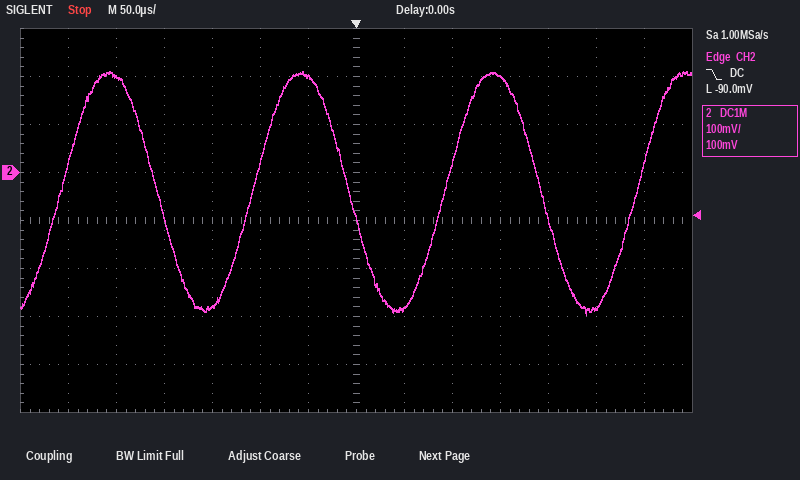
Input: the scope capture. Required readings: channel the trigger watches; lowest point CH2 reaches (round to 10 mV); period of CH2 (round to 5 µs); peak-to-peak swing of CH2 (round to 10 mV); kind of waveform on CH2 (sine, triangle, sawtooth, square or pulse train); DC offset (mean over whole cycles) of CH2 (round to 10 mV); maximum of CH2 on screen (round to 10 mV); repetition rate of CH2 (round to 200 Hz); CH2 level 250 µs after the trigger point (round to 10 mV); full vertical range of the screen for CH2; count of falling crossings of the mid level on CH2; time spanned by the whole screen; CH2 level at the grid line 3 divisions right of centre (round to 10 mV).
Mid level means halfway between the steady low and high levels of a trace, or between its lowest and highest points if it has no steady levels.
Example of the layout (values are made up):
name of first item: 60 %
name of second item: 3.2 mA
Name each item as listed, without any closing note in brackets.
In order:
channel the trigger watches: CH2
lowest point CH2 reaches: -300 mV
period of CH2: 200 µs
peak-to-peak swing of CH2: 510 mV
kind of waveform on CH2: sine
DC offset (mean over whole cycles) of CH2: -40 mV
maximum of CH2 on screen: 210 mV
repetition rate of CH2: 5.0 kHz
CH2 level 250 µs after the trigger point: -280 mV
full vertical range of the screen for CH2: 800 mV
count of falling crossings of the mid level on CH2: 3
time spanned by the whole screen: 700 µs
CH2 level at the grid line 3 divisions right of centre: 200 mV
